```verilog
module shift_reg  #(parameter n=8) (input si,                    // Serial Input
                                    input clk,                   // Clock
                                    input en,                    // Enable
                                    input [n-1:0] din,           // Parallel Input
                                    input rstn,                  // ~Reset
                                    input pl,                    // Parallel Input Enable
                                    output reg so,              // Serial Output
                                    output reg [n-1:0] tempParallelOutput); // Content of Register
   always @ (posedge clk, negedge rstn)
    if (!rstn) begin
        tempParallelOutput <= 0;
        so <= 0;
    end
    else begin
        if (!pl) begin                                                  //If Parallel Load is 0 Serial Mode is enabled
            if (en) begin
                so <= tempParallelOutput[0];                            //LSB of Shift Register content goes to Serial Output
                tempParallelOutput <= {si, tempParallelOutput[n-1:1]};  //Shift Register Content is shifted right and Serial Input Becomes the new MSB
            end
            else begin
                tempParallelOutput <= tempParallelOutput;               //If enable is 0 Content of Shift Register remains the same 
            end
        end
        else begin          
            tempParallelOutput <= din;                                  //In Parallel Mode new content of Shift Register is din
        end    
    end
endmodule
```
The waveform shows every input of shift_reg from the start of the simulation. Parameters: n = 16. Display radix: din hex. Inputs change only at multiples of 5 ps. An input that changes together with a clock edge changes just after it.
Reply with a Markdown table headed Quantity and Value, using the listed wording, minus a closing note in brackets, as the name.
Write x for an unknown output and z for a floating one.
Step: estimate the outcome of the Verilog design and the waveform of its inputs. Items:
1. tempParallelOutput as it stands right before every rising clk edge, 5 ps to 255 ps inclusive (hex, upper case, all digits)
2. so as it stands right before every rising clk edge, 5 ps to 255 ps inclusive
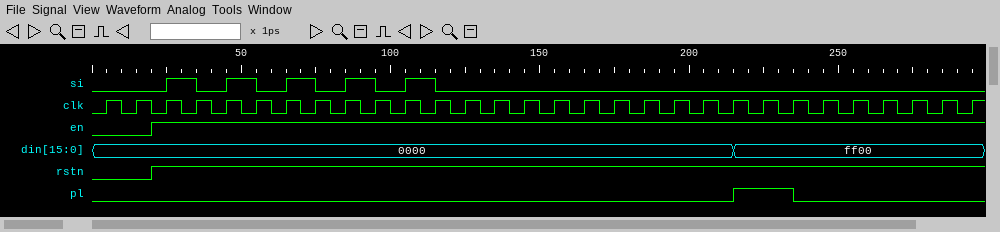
| Quantity | Value |
|---|---|
| tempParallelOutput as it stands right before every rising clk edge, 5 ps to 255 ps inclusive | 0000, 0000, 0000, 0000, 8000, 4000, A000, 5000, A800, 5400, AA00, 5500, AA80, 5540, 2AA0, 1550, 0AA8, 0554, 02AA, 0155, 00AA, 0055, 002A, FF00, FF00, 7F80 |
| so as it stands right before every rising clk edge, 5 ps to 255 ps inclusive | 0 0 0 0 0 0 0 0 0 0 0 0 0 0 0 0 0 0 0 0 1 0 1 1 1 0 |
